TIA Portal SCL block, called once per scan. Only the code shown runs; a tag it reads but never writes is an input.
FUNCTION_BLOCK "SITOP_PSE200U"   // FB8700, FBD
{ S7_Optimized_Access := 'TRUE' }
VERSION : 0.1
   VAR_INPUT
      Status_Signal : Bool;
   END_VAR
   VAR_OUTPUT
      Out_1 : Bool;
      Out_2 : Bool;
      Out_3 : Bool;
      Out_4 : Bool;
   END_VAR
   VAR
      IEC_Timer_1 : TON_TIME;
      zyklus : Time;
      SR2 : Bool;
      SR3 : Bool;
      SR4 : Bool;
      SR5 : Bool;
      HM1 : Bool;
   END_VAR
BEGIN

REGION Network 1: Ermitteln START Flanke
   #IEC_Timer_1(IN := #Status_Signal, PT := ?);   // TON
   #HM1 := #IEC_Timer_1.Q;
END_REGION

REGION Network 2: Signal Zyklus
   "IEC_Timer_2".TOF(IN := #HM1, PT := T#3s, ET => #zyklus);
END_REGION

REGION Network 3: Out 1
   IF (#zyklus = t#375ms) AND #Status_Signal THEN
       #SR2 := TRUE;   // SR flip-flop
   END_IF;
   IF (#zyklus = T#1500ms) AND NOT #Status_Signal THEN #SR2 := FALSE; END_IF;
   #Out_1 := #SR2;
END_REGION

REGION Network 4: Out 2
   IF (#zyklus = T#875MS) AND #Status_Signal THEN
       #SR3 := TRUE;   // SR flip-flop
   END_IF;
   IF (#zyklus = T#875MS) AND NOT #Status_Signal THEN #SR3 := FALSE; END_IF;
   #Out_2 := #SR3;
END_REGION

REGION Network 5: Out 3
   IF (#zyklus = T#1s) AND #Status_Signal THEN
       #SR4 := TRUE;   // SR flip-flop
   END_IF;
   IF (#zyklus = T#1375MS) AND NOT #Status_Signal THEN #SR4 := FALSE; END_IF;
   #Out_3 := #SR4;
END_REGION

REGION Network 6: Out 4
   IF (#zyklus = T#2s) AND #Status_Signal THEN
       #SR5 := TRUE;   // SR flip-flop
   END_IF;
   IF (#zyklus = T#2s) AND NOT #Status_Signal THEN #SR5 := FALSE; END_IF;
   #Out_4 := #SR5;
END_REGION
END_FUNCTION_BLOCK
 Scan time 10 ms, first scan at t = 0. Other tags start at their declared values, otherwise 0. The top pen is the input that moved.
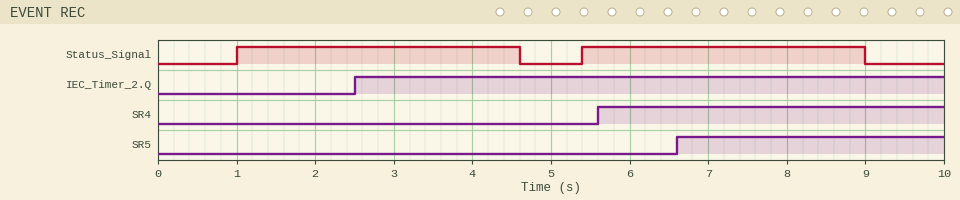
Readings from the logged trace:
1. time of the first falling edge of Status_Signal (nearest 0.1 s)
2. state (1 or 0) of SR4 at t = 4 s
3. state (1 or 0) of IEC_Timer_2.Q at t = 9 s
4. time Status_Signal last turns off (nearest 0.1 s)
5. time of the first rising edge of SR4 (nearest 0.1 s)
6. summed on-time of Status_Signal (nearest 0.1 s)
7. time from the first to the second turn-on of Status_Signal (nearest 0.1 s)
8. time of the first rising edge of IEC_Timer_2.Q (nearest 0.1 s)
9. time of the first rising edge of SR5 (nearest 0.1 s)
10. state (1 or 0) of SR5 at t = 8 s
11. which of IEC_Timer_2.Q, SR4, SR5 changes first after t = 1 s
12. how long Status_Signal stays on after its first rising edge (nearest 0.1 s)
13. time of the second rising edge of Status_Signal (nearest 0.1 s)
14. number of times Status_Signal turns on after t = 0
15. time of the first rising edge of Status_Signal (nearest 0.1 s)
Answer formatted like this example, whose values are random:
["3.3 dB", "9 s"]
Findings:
["4.6 s", "0", "1", "9.0 s", "5.6 s", "7.2 s", "4.4 s", "2.5 s", "6.6 s", "1", "IEC_Timer_2.Q", "3.6 s", "5.4 s", "2", "1.0 s"]
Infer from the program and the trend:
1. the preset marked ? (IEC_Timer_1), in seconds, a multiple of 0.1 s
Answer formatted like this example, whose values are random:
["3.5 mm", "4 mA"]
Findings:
["1.5 s"]
